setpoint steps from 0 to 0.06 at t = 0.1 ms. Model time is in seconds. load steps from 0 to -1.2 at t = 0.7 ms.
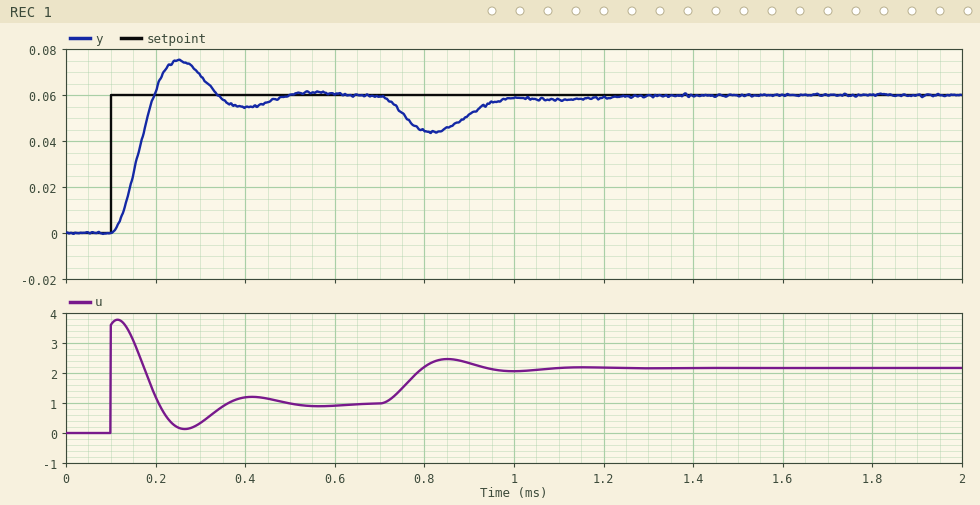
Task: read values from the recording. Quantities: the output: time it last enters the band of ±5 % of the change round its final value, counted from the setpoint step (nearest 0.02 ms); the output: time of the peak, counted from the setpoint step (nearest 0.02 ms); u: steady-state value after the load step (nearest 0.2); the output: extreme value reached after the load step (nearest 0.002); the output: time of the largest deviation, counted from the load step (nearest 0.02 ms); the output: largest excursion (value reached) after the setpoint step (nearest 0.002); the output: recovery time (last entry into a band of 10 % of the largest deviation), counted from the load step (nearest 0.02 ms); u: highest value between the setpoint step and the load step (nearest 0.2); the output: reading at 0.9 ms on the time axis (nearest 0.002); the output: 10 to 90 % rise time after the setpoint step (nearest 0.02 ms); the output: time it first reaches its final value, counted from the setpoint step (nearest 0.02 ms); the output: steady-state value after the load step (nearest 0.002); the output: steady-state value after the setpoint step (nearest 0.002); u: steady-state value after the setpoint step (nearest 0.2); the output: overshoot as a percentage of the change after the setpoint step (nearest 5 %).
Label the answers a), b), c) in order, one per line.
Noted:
a) 0.36 ms
b) 0.16 ms
c) 2.2
d) 0.044
e) 0.12 ms
f) 0.076
g) 0.46 ms
h) 3.8
i) 0.052
j) 0.06 ms
k) 0.10 ms
l) 0.060
m) 0.060
n) 1.0
o) 25 %
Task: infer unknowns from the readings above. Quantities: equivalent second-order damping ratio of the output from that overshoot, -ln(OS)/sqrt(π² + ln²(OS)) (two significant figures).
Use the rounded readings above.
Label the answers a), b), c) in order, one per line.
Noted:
a) 0.40
